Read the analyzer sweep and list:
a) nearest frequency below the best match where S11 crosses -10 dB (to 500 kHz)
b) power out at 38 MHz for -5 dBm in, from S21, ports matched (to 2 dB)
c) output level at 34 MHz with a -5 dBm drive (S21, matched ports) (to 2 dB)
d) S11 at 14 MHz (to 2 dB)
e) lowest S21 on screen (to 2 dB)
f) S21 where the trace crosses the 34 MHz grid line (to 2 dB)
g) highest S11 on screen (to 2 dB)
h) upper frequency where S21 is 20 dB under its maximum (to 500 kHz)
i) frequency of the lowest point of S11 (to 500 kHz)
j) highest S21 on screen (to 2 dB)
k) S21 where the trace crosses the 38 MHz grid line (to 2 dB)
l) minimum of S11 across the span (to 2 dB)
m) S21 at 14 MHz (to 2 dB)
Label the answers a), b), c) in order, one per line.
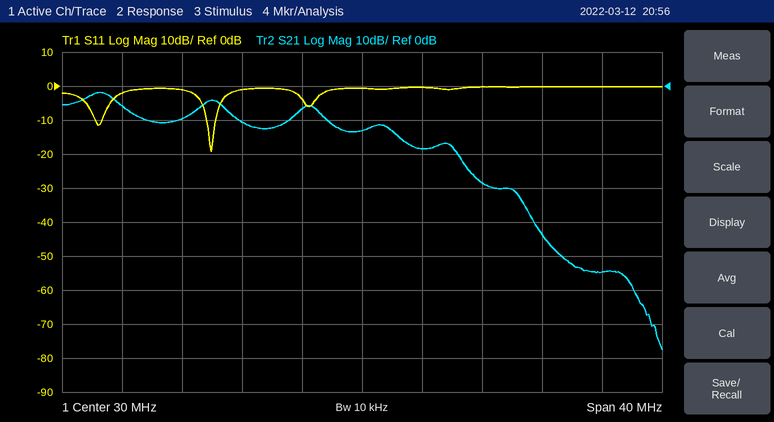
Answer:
a) 19.5 MHz
b) -34 dBm
c) -24 dBm
d) -2 dB
e) -78 dB
f) -18 dB
g) 0 dB
h) 36.5 MHz
i) 20.0 MHz
j) -2 dB
k) -28 dB
l) -20 dB
m) -6 dB
